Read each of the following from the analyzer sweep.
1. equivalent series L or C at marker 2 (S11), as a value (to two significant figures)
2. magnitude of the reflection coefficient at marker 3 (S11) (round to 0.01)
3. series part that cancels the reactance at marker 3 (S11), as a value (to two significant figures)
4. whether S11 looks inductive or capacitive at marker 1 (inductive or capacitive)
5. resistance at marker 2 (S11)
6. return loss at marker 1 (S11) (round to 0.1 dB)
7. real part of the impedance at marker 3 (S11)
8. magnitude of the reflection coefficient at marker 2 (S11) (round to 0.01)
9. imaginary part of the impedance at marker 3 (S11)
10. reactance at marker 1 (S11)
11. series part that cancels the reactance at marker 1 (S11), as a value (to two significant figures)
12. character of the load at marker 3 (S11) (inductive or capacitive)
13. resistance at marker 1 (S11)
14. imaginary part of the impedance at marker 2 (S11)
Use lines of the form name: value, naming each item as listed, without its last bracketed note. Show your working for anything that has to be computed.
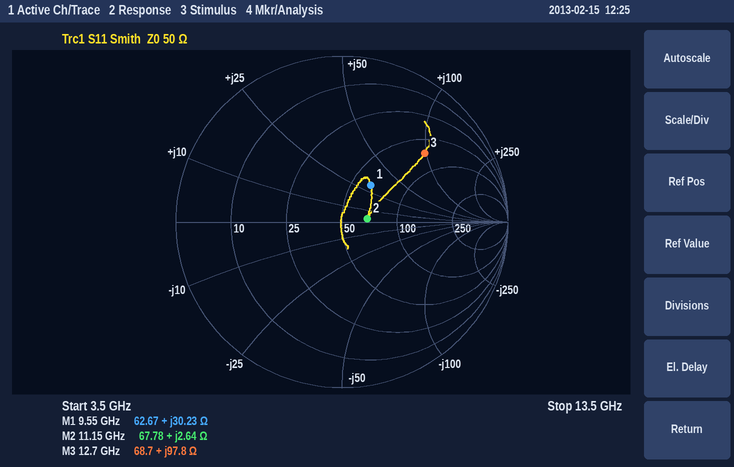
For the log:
equivalent series L or C at marker 2 (S11), as a value: L = 2.64 Ω/(2π × 11.15 GHz) ≈ 38 pH
magnitude of the reflection coefficient at marker 3 (S11): 0.65
series part that cancels the reactance at marker 3 (S11), as a value: C = 1/(2π × 12.7 GHz × 97.8 Ω) ≈ 128 fF, so 130 fF to two significant figures
whether S11 looks inductive or capacitive at marker 1: inductive
resistance at marker 2: 67.78 Ω
return loss at marker 1 (S11): 11.0 dB
real part of the impedance at marker 3: 68.7 Ω
magnitude of the reflection coefficient at marker 2 (S11): 0.15
imaginary part of the impedance at marker 3: +97.8 Ω
reactance at marker 1: +30.23 Ω
series part that cancels the reactance at marker 1 (S11), as a value: C = 1/(2π × 9.55 GHz × 30.23 Ω) ≈ 551 fF, so 550 fF to two significant figures
character of the load at marker 3 (S11): inductive
resistance at marker 1: 62.67 Ω
imaginary part of the impedance at marker 2: +2.64 Ω
